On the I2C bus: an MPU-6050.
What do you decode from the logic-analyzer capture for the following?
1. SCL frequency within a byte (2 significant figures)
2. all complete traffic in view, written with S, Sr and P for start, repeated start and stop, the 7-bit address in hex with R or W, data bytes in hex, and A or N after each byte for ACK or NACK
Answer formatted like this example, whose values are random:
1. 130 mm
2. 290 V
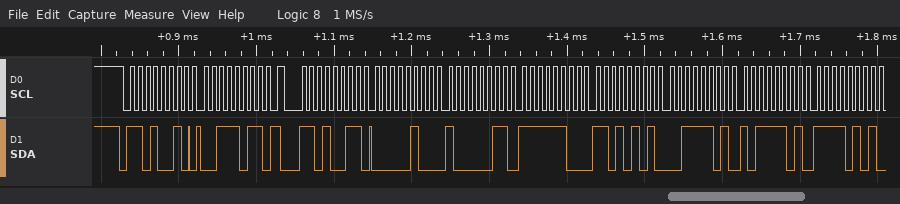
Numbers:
1. 100 kHz
2. S 69W A 3B A Sr 69R A 04 A 83 A FC A D5 A 3D A BD A F5 A
